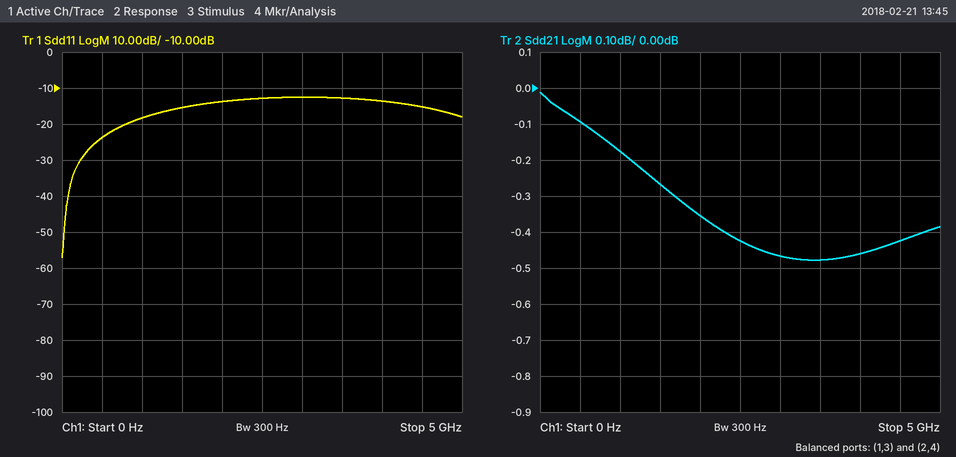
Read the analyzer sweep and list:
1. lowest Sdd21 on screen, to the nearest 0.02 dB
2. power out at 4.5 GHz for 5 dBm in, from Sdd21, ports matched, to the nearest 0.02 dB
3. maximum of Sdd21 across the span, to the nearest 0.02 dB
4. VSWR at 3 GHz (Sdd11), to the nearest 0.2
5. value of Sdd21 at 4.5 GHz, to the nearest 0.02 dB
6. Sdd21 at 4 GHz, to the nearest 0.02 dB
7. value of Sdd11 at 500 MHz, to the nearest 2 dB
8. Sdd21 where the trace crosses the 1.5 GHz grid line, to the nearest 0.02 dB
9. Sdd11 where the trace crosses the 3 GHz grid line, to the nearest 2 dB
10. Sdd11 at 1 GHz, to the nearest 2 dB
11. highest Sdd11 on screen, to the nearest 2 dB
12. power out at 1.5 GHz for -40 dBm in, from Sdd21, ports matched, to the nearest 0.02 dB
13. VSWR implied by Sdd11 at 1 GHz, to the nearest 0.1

-0.48 dB
4.58 dBm
-0.02 dB
1.6
-0.42 dB
-0.46 dB
-24 dB
-0.26 dB
-12 dB
-18 dB
-12 dB
-40.26 dBm
1.3
